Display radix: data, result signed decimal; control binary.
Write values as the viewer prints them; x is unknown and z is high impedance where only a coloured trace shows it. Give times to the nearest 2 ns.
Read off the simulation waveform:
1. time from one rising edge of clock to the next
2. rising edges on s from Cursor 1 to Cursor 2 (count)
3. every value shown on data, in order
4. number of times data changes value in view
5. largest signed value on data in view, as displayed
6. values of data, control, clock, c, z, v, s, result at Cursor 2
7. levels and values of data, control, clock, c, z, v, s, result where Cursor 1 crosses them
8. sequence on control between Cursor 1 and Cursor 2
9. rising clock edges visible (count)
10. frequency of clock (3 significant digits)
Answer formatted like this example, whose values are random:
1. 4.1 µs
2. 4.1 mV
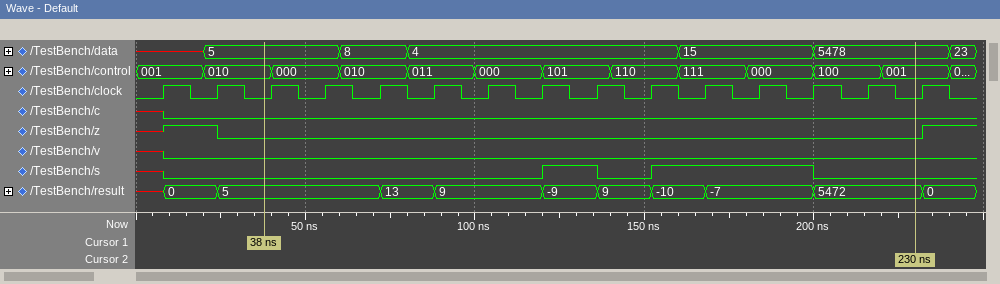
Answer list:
1. 16 ns
2. 2
3. x, 5, 8, 4, 15, 5478, 23
4. 6
5. 5478
6. data=5478, control=001, clock=0, c=0, z=0, v=0, s=0, result=5472
7. data=5, control=010, clock=0, c=0, z=0, v=0, s=0, result=5
8. 010, 000, 010, 011, 000, 101, 110, 111, 000, 100, 001
9. 15
10. 62.5 MHz
